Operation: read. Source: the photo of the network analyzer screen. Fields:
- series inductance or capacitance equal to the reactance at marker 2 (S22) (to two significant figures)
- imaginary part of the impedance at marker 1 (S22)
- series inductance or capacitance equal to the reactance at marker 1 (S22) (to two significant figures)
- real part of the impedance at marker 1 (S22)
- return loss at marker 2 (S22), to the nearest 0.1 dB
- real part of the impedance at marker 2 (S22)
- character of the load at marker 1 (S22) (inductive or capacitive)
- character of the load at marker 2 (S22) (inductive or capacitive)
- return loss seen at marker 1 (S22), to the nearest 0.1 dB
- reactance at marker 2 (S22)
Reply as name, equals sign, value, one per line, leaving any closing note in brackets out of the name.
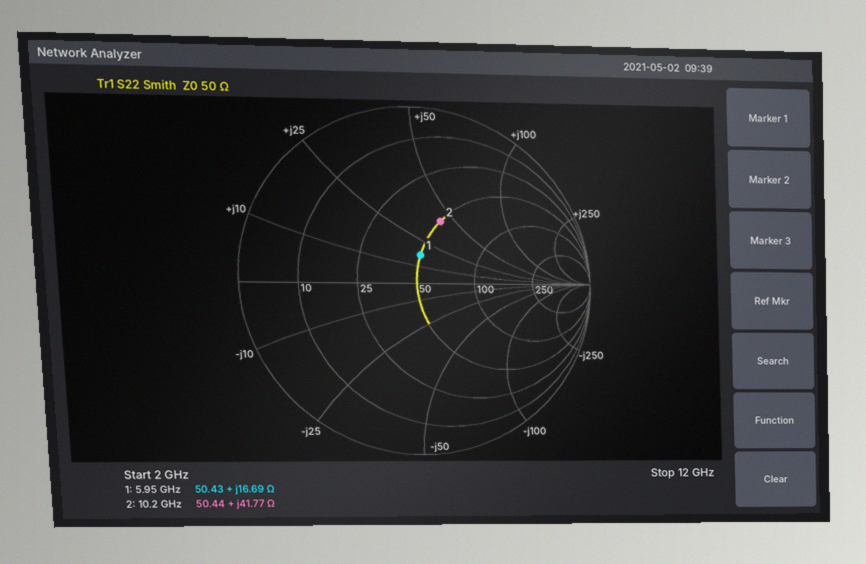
series inductance or capacitance equal to the reactance at marker 2 (S22) = 650 pH
imaginary part of the impedance at marker 1 = +16.69 Ω
series inductance or capacitance equal to the reactance at marker 1 (S22) = 450 pH
real part of the impedance at marker 1 = 50.43 Ω
return loss at marker 2 (S22), to the nearest 0.1 dB = 8.3 dB
real part of the impedance at marker 2 = 50.44 Ω
character of the load at marker 1 (S22) = inductive
character of the load at marker 2 (S22) = inductive
return loss seen at marker 1 (S22), to the nearest 0.1 dB = 15.7 dB
reactance at marker 2 = +41.77 Ω
